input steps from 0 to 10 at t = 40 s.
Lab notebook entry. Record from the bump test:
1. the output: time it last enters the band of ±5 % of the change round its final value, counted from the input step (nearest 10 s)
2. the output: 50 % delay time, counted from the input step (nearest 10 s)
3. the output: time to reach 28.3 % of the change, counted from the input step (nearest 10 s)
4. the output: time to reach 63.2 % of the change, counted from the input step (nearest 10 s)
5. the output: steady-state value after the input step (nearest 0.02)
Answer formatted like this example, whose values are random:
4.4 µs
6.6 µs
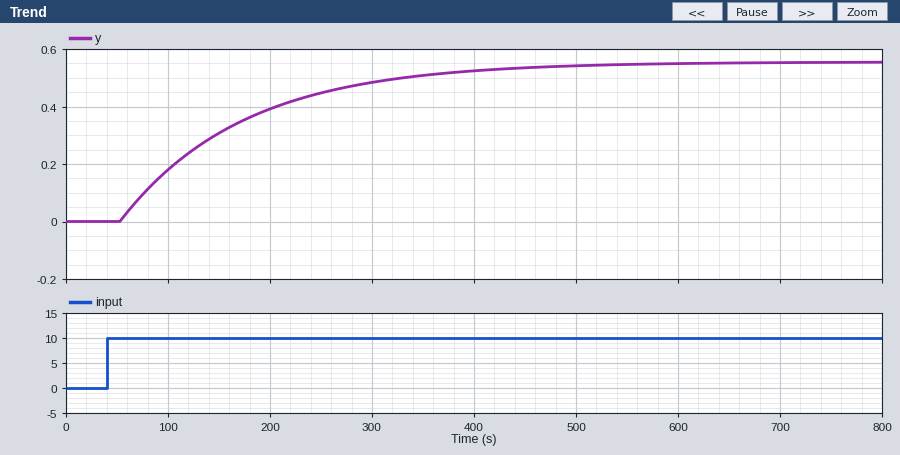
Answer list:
370 s
100 s
50 s
130 s
0.56
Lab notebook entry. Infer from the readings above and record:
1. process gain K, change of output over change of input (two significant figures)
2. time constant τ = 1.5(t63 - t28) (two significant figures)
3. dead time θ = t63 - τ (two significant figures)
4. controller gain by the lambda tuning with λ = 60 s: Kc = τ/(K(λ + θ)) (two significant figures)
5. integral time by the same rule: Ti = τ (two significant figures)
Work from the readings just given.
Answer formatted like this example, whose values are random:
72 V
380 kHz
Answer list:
0.056
120 s
10 s
31
120 s
